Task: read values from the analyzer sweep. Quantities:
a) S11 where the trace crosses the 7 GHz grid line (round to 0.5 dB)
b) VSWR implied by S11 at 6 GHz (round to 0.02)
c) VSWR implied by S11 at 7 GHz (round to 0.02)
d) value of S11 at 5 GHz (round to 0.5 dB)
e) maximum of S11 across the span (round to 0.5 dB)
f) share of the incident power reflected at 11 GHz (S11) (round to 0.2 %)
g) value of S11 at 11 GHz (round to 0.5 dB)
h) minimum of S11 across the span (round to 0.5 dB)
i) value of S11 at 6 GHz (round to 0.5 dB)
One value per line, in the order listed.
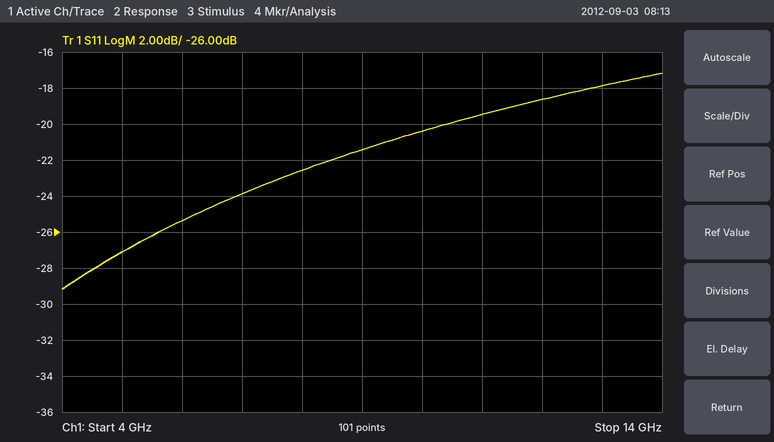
-24.0 dB
1.12
1.14
-27.0 dB
-17.0 dB
1.2 %
-19.5 dB
-29.0 dB
-25.5 dB
